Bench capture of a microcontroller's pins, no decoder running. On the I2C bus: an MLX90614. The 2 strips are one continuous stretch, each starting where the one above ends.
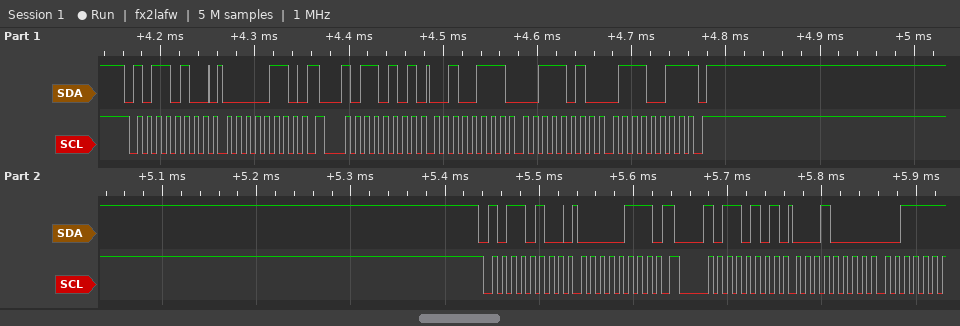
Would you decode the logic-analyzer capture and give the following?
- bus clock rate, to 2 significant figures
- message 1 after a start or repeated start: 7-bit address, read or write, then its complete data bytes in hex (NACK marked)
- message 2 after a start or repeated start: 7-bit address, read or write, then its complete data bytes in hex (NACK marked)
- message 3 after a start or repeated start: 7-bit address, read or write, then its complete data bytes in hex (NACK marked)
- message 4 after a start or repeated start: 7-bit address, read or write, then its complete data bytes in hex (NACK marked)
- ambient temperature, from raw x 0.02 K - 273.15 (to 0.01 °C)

100 kHz
0x5A write: 06
0x5A read: 27 3A 73 NACK
0x5A write: 07
0x5A read: 10
24.59 °C
